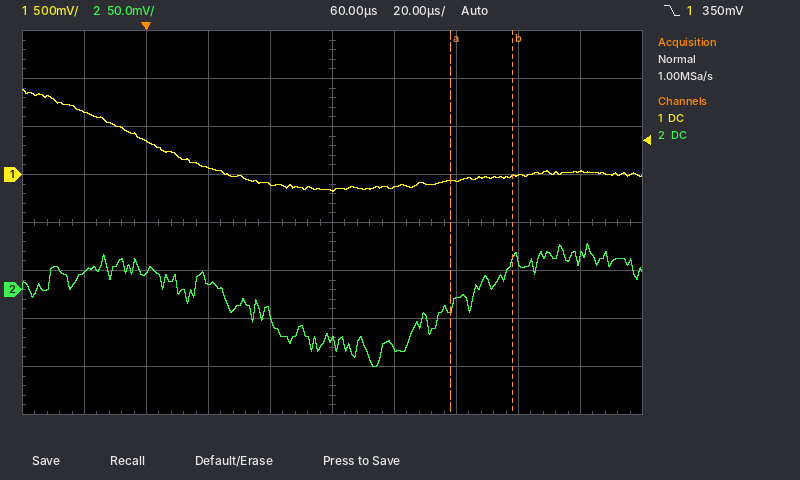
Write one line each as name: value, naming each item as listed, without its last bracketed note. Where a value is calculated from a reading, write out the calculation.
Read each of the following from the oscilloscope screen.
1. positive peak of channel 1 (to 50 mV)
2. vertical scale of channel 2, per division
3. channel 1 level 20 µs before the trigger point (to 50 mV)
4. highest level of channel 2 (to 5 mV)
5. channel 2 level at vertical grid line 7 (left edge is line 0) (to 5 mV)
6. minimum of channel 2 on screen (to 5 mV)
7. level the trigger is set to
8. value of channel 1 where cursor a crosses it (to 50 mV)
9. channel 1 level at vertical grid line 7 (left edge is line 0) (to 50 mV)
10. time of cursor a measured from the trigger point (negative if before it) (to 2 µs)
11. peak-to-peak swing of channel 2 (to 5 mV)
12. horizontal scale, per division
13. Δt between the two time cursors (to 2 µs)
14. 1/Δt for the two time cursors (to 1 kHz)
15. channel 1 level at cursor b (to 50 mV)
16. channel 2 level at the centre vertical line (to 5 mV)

positive peak of channel 1: 900 mV
vertical scale of channel 2, per division: 50 mV
channel 1 level 20 µs before the trigger point: 650 mV
highest level of channel 2: 50 mV
channel 2 level at vertical grid line 7 (left edge is line 0): -10 mV
minimum of channel 2 on screen: -80 mV
level the trigger is set to: 350 mV
value of channel 1 where cursor a crosses it: -50 mV
channel 1 level at vertical grid line 7 (left edge is line 0): -50 mV
time of cursor a measured from the trigger point (negative if before it): +98 µs
peak-to-peak swing of channel 2: 50 mV − (-80 mV) = 130 mV
horizontal scale, per division: 20 µs
Δt between the two time cursors: 20 µs
1/Δt for the two time cursors: 1 / 20 µs ≈ 50 kHz
channel 1 level at cursor b: 0 mV
channel 2 level at the centre vertical line: -55 mV
